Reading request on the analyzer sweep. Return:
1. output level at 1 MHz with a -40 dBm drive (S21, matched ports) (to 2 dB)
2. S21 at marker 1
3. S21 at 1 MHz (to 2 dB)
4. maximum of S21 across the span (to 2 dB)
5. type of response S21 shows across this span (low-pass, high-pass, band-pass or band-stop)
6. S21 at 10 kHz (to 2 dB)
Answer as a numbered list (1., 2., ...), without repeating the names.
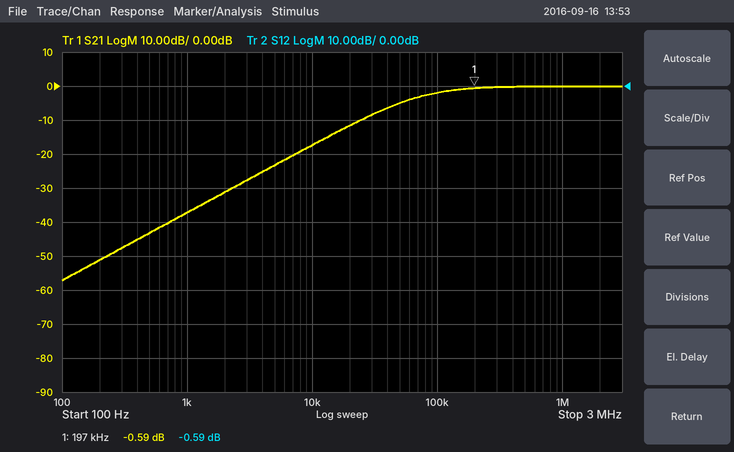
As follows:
1. -40 dBm
2. -0.59 dB
3. 0 dB
4. 0 dB
5. high-pass
6. -18 dB
